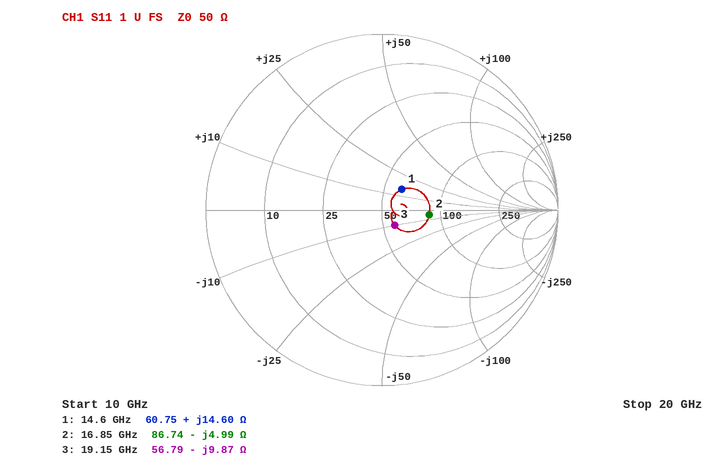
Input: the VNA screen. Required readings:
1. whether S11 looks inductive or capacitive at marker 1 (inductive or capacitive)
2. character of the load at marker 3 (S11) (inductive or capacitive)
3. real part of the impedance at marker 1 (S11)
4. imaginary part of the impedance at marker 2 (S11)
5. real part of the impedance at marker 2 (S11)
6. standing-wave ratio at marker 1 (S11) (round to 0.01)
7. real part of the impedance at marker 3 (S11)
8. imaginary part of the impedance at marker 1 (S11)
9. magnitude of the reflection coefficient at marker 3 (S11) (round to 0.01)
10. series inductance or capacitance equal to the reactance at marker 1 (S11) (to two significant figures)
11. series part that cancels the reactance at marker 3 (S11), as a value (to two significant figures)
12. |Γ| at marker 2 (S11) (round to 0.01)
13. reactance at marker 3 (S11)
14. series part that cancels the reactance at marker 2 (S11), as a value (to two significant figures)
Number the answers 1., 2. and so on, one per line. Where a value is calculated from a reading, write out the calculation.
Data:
1. inductive
2. capacitive
3. 60.75 Ω
4. -4.99 Ω
5. 86.74 Ω
6. 1.39
7. 56.79 Ω
8. +14.60 Ω
9. 0.11
10. L = 14.6 Ω/(2π × 14.6 GHz) ≈ 159 pH, so 160 pH to two significant figures
11. L = 9.87 Ω/(2π × 19.15 GHz) ≈ 82 pH
12. 0.27
13. -9.87 Ω
14. L = 4.99 Ω/(2π × 16.85 GHz) ≈ 47 pH
